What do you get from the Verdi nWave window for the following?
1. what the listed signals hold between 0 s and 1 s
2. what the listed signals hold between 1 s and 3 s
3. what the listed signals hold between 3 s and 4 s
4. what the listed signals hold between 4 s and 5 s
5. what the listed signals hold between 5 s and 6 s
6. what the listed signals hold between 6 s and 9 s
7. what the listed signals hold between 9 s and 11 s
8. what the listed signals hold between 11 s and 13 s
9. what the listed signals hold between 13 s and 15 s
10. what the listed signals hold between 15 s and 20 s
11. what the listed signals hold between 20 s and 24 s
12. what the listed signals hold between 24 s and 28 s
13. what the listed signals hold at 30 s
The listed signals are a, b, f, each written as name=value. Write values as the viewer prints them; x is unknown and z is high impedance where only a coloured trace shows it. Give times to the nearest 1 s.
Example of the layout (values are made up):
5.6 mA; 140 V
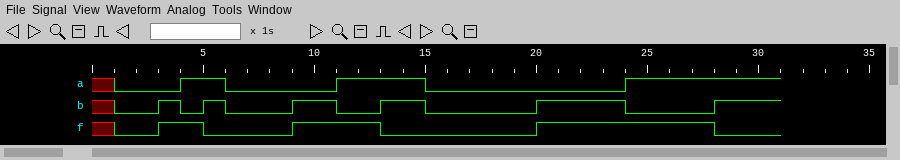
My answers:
a=x, b=x, f=x; a=0, b=0, f=0; a=0, b=1, f=1; a=1, b=0, f=1; a=1, b=1, f=0; a=0, b=0, f=0; a=0, b=1, f=1; a=1, b=0, f=1; a=1, b=1, f=0; a=0, b=0, f=0; a=0, b=1, f=1; a=1, b=0, f=1; a=1, b=1, f=0
